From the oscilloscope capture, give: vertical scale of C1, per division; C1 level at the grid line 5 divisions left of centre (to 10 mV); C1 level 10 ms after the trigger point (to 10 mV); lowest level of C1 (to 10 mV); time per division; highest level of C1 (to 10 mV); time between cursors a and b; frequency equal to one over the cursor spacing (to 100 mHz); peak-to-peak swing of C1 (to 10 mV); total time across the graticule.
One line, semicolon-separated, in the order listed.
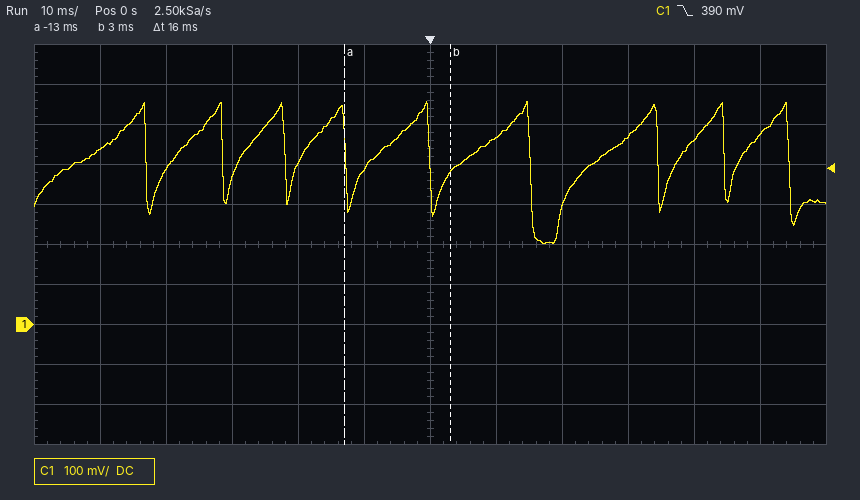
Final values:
100 mV; 440 mV; 470 mV; 200 mV; 10 ms; 560 mV; 16 ms; 62.5 Hz; 360 mV; 120 ms
